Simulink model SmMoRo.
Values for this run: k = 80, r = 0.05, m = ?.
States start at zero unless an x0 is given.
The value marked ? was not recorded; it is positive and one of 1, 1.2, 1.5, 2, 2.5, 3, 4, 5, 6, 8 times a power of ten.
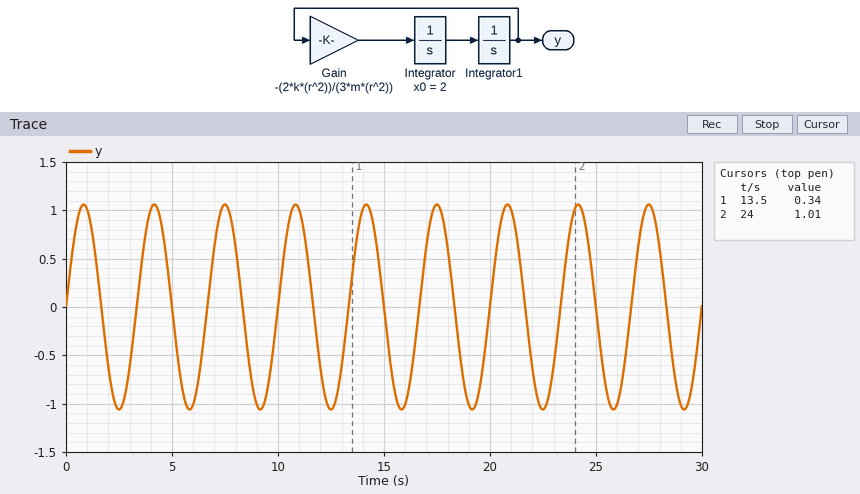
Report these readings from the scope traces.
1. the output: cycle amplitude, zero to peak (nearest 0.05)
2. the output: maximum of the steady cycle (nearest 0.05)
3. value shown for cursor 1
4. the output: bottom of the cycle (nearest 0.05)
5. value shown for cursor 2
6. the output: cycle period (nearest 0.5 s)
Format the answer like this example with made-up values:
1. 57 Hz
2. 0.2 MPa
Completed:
1. 1.05
2. 1.05
3. 0.34
4. -1.05
5. 1.01
6. 3.5 s
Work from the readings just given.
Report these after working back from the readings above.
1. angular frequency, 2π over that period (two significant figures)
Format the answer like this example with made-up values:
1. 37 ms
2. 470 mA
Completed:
1. 1.8 rad/s
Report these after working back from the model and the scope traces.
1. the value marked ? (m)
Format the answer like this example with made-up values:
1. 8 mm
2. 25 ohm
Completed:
1. 15
